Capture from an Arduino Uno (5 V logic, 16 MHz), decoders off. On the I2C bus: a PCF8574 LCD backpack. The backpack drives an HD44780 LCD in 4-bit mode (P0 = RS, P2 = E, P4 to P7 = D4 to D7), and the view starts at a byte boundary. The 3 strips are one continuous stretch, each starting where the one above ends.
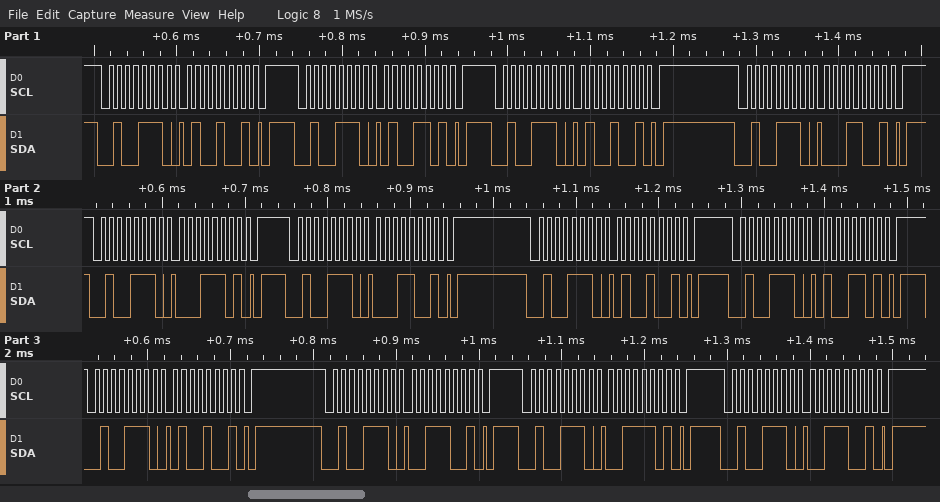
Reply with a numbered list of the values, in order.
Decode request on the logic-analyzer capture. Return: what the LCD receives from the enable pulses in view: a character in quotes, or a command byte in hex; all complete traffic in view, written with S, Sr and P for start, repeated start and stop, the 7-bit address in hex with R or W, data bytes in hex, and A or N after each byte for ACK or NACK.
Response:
1. 'A' 'C'
2. S 27W A 49 A P S 27W A 4D A P S 27W A 49 A P S 27W A 19 A P S 27W A 1D A P S 27W A 19 A P S 27W A 49 A P S 27W A 4D A P S 27W A 49 A P S 27W A 39 A P S 27W A 3D A P S 27W A 39 A P
